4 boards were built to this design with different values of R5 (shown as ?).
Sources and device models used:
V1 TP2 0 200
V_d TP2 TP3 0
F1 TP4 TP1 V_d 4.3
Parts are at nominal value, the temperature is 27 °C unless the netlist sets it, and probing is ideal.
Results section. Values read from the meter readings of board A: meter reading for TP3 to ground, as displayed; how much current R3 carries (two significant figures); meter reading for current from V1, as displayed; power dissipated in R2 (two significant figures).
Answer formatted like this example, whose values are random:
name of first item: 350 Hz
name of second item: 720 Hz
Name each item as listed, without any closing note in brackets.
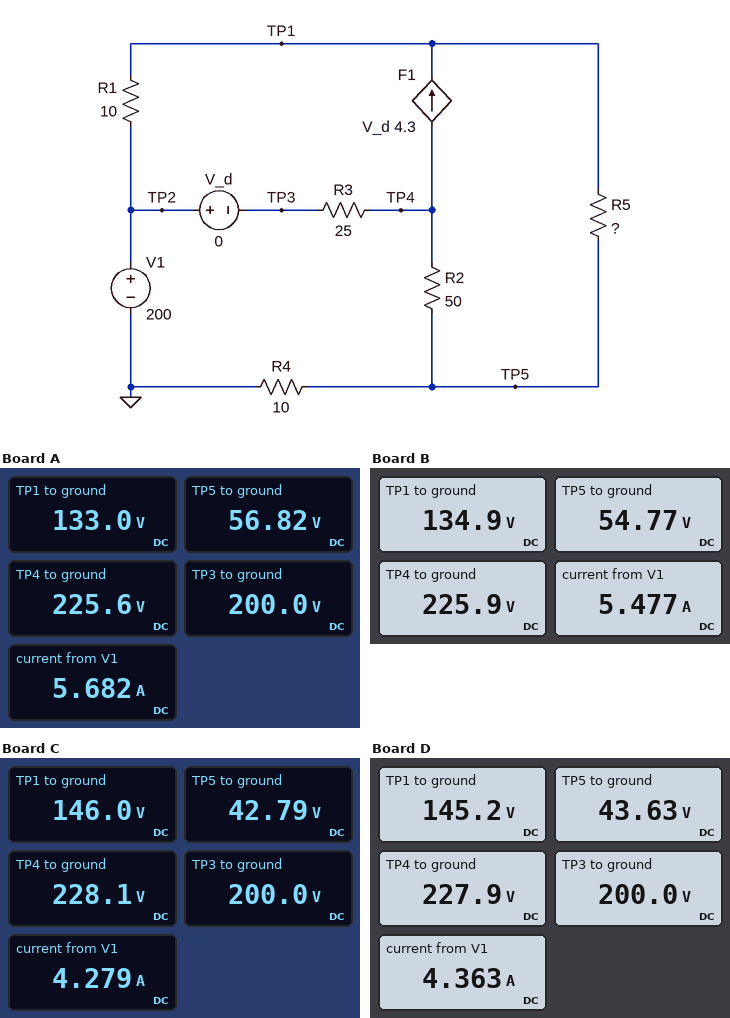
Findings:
meter reading for TP3 to ground, as displayed: 200.0 V
how much current R3 carries: 1.0 A
meter reading for current from V1, as displayed: 5.682 A
power dissipated in R2: 570 W
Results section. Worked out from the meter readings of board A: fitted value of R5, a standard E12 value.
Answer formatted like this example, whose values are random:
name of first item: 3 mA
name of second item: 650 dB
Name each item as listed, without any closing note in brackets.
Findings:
fitted value of R5, a standard E12 value: 33 Ω
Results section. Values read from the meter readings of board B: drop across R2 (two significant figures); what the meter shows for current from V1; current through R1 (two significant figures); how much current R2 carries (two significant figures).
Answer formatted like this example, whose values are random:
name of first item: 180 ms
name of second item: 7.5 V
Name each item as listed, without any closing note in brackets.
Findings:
drop across R2: 170 V
what the meter shows for current from V1: 5.477 A
current through R1: 6.5 A
how much current R2 carries: 3.4 A
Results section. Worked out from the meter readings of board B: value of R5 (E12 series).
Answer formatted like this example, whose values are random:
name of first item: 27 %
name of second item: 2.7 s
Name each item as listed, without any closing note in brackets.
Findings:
value of R5: 39 Ω
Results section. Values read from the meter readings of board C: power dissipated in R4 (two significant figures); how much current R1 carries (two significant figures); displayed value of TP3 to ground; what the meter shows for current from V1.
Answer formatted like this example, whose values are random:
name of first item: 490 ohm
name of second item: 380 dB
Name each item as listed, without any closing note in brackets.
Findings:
power dissipated in R4: 180 W
how much current R1 carries: 5.4 A
displayed value of TP3 to ground: 200.0 V
what the meter shows for current from V1: 4.279 A
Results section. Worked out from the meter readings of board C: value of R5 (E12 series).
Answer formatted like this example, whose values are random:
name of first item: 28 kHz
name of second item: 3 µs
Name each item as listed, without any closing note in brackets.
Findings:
value of R5: 180 Ω
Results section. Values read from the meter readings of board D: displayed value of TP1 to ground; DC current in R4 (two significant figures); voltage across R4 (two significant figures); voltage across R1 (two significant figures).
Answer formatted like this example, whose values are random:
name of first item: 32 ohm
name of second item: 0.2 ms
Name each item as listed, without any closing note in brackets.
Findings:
displayed value of TP1 to ground: 145.2 V
DC current in R4: 4.4 A
voltage across R4: 44 V
voltage across R1: 55 V
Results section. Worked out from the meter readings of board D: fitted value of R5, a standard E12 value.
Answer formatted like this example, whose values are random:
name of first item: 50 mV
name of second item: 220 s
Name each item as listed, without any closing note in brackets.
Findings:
fitted value of R5, a standard E12 value: 150 Ω
